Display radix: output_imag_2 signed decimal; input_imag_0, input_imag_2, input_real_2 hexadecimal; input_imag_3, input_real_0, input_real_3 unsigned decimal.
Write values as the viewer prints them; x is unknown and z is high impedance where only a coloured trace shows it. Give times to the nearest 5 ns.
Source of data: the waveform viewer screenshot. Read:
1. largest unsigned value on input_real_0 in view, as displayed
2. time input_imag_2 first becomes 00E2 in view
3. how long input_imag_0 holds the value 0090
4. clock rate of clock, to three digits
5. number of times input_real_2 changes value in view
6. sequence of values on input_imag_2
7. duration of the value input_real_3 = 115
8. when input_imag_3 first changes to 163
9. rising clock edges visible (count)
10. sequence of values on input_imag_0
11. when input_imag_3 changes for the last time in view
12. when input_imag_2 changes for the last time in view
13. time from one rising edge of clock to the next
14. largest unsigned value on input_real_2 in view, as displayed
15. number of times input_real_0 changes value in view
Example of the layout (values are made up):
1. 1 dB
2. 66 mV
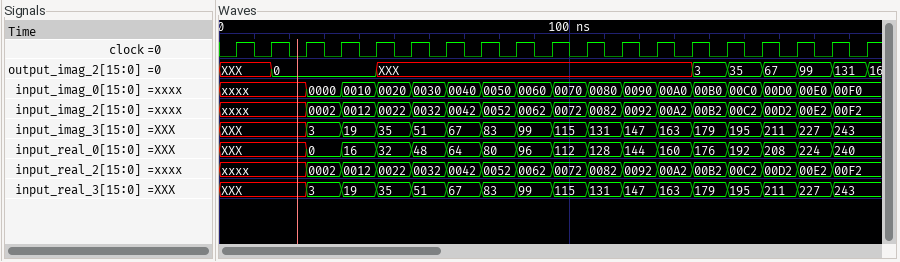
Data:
1. 240
2. 165 ns
3. 10 ns
4. 100 MHz
5. 16
6. xxxx, 0002, 0012, 0022, 0032, 0042, 0052, 0062, 0072, 0082, 0092, 00A2, 00B2, 00C2, 00D2, 00E2, 00F2
7. 10 ns
8. 125 ns
9. 19
10. xxxx, 0000, 0010, 0020, 0030, 0040, 0050, 0060, 0070, 0080, 0090, 00A0, 00B0, 00C0, 00D0, 00E0, 00F0
11. 175 ns
12. 175 ns
13. 10 ns
14. 00F2
15. 16
